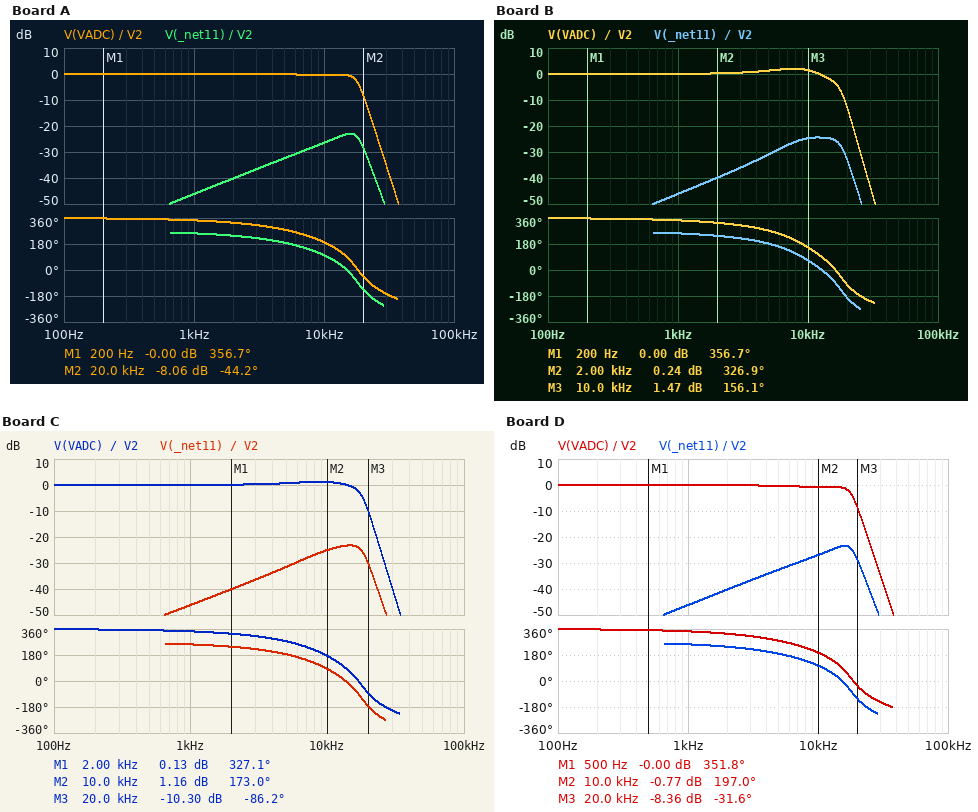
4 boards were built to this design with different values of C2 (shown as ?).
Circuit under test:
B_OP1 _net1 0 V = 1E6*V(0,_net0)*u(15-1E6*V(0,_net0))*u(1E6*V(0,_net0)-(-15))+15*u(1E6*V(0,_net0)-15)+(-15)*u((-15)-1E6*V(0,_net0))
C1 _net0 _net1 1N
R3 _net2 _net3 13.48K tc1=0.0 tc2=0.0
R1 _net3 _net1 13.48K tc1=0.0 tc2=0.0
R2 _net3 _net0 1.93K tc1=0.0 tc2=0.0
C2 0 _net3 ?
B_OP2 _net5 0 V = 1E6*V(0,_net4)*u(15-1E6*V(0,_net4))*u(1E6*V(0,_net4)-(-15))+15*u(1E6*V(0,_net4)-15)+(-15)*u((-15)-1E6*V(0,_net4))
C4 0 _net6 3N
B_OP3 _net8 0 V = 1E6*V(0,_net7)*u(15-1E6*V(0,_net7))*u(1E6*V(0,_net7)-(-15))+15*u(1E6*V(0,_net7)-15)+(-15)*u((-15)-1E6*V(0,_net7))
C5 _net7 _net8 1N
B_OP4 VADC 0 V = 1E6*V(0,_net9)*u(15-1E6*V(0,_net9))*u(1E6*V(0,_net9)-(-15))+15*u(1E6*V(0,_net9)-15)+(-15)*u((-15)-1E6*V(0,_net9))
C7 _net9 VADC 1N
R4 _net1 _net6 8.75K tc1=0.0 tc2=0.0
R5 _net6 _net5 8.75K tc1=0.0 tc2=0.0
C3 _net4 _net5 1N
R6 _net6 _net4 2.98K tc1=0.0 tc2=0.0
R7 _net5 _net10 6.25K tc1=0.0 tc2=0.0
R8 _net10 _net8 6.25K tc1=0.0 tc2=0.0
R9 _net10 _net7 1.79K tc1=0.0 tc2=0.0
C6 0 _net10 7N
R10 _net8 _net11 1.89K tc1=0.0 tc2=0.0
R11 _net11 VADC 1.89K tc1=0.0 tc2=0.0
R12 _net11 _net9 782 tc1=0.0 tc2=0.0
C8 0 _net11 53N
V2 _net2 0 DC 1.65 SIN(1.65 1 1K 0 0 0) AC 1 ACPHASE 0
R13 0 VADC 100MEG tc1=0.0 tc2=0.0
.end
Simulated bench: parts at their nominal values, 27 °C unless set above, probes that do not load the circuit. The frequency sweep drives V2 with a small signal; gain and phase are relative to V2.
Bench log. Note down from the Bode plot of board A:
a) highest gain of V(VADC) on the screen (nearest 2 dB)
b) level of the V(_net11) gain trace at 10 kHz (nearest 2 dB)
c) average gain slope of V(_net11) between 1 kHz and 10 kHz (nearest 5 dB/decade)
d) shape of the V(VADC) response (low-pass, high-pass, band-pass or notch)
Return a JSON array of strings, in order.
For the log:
["0 dB", "-26 dB", "20 dB/decade", "low-pass"]
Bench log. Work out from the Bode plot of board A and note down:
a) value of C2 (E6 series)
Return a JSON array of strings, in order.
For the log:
["2.2 nF"]
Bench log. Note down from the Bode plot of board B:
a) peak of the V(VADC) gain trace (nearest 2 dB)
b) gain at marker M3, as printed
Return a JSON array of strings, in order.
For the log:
["2 dB", "1.47 dB"]
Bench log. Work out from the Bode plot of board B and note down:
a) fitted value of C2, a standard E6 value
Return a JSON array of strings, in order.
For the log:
["10 nF"]
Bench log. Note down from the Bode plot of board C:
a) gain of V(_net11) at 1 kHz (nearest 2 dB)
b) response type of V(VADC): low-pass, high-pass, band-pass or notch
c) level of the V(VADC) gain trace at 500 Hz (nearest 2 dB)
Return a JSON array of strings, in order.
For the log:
["-46 dB", "low-pass", "0 dB"]
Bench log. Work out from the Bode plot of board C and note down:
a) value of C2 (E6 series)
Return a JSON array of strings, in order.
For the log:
["6.8 nF"]
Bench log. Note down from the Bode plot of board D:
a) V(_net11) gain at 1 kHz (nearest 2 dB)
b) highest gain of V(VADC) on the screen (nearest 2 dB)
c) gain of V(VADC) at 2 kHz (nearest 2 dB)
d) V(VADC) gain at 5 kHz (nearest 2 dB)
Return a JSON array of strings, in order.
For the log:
["-46 dB", "0 dB", "0 dB", "0 dB"]
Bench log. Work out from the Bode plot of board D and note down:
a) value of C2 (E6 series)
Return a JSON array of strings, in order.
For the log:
["1 nF"]
